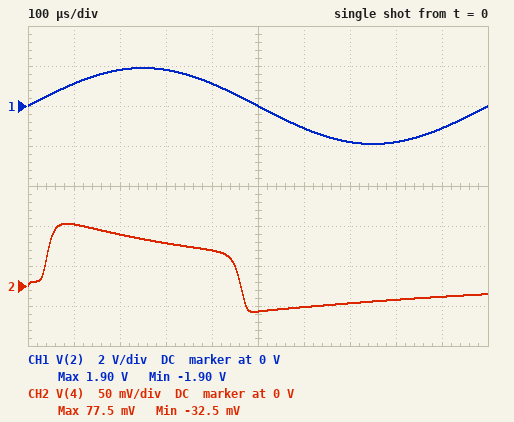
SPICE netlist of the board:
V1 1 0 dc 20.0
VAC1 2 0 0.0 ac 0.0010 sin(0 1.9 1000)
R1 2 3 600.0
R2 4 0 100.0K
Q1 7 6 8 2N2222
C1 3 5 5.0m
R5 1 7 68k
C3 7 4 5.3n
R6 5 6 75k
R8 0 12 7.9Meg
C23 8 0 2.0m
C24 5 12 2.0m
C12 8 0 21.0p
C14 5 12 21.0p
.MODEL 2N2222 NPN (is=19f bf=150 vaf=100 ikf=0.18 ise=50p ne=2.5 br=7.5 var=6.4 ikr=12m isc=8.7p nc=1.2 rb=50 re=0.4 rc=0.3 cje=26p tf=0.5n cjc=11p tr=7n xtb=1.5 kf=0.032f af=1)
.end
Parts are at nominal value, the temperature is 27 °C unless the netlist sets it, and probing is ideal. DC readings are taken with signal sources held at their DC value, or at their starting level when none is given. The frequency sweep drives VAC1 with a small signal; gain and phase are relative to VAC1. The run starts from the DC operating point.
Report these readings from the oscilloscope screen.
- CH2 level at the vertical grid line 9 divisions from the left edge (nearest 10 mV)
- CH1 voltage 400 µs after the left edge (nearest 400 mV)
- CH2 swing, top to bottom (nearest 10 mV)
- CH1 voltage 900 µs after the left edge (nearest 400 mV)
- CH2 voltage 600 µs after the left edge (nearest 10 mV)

-10 mV
1.2 V
110 mV
-1.2 V
-30 mV
